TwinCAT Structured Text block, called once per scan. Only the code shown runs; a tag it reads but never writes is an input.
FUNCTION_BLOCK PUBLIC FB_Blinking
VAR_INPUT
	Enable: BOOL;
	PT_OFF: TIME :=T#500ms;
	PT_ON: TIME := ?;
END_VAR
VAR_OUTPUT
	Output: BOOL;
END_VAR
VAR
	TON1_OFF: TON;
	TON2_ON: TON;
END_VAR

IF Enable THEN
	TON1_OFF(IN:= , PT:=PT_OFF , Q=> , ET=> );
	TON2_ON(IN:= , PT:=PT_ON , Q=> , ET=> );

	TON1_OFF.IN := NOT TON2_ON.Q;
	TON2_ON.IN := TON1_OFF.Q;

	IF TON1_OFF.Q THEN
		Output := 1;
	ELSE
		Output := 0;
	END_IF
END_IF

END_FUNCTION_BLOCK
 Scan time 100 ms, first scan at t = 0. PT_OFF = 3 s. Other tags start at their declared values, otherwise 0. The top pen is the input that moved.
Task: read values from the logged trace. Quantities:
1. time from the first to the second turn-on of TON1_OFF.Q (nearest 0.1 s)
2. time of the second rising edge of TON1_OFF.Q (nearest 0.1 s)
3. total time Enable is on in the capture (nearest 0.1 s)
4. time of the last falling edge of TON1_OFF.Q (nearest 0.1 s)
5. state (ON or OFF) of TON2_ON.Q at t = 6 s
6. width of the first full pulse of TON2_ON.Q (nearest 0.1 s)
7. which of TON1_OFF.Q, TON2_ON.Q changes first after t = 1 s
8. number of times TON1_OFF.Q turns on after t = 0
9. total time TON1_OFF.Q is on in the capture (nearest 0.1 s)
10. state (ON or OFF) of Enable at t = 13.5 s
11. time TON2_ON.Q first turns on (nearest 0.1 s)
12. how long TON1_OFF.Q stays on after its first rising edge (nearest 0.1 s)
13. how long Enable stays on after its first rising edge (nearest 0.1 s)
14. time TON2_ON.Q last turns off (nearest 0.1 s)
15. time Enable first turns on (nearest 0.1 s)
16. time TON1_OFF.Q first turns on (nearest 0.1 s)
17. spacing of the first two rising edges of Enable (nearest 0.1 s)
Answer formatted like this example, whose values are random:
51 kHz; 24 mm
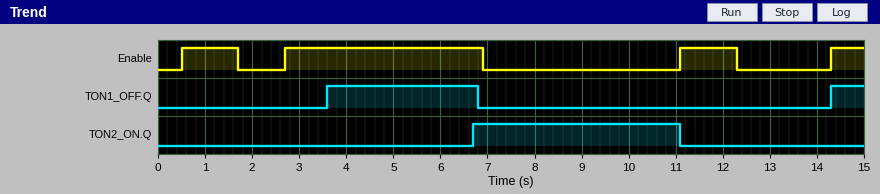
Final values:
10.7 s; 14.3 s; 7.3 s; 6.8 s; OFF; 4.4 s; TON1_OFF.Q; 2; 3.9 s; OFF; 6.7 s; 3.2 s; 1.2 s; 11.1 s; 0.5 s; 3.6 s; 2.2 s
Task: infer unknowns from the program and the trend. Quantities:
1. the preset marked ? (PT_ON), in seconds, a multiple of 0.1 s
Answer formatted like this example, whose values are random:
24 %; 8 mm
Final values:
3.0 s
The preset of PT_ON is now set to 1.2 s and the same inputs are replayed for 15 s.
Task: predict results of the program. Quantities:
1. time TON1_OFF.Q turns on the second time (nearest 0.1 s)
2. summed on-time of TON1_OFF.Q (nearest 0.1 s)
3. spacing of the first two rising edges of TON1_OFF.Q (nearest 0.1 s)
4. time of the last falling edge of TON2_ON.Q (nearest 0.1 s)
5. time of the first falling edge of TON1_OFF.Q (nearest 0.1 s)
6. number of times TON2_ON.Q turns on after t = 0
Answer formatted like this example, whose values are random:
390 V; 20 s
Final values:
11.1 s; 4.7 s; 7.5 s; 14.5 s; 5.0 s; 2
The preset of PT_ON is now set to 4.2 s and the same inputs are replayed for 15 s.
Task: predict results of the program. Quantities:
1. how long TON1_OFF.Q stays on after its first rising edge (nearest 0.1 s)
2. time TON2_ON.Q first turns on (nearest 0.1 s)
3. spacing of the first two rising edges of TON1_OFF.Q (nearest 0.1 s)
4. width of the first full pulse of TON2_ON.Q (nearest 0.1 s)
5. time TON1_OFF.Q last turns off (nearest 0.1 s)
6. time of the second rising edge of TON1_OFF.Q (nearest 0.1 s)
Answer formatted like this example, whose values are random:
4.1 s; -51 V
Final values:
7.6 s; 11.1 s; 10.8 s; 0.2 s; 11.2 s; 14.4 s
